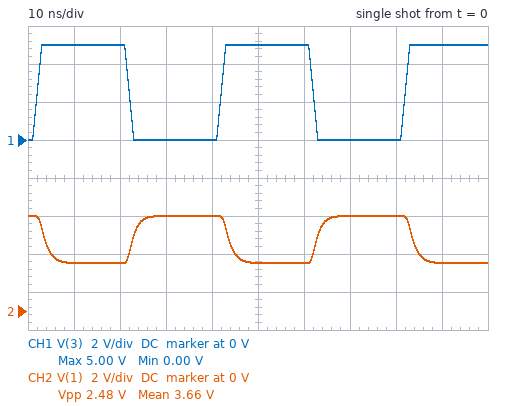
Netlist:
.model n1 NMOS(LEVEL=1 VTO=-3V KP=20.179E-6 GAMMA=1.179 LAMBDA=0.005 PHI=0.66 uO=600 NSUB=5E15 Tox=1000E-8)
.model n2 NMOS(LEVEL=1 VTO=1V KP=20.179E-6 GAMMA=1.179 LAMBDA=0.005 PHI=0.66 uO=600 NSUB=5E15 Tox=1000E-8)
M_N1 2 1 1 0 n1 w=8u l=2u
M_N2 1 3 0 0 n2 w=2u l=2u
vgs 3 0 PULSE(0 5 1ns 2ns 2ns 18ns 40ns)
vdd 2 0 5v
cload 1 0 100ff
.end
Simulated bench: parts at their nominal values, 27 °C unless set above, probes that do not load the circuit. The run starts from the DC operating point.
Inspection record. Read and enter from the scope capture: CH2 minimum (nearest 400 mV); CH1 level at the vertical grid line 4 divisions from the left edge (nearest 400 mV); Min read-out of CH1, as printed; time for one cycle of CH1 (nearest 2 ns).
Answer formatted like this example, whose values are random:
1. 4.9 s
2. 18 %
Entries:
1. 2.4 V
2. 0 V
3. 0.00 V
4. 40 ns
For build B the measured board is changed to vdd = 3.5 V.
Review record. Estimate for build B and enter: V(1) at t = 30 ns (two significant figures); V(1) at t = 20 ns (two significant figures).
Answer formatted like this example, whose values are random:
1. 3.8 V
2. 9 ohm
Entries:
1. 3.5 V
2. 2.3 V
